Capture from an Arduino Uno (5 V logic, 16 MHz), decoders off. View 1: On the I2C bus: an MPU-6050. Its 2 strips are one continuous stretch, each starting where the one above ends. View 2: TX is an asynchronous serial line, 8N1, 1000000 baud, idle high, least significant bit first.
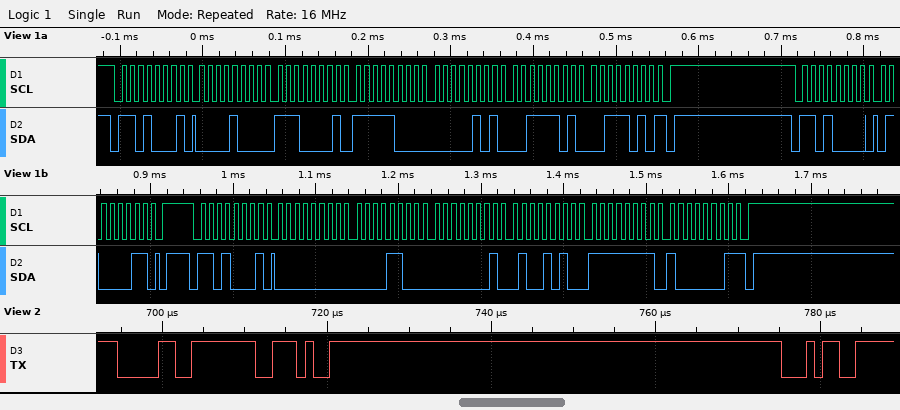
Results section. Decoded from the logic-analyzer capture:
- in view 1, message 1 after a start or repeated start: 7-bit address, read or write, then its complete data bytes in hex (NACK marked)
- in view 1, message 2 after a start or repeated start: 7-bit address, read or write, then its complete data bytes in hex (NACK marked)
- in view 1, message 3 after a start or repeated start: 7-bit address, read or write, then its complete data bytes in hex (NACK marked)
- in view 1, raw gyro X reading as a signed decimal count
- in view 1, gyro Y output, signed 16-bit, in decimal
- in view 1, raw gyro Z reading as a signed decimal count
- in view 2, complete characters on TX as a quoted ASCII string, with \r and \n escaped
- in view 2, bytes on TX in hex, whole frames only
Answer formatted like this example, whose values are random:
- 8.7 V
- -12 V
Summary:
- 0x68 read: 08 E1 F8 05 3D 3A NACK
- 0x68 write: 43
- 0x68 read: 00 0C 01 4A FF 81 NACK
- 12
- 330
- -127
- "0.4"
- 30 2E 34
